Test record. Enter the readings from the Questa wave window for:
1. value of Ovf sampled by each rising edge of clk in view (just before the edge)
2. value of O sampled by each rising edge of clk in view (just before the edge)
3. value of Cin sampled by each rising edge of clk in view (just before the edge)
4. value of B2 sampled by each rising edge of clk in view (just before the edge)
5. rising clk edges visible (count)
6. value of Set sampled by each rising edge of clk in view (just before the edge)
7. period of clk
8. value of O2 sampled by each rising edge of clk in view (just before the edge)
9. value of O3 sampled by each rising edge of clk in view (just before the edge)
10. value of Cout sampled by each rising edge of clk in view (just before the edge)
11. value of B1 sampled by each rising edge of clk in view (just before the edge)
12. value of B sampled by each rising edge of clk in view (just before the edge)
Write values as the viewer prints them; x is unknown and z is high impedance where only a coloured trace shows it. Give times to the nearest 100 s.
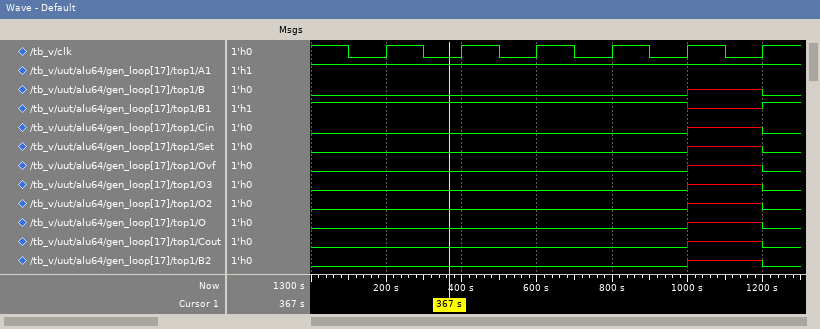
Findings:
0 0 0 0 0 x
0 0 0 0 0 x
0 0 0 0 0 x
0 0 0 0 0 x
6
0 0 0 0 0 x
200 s
0 0 0 0 0 x
0 0 0 0 0 x
0 0 0 0 0 x
1 1 1 1 1 x
0 0 0 0 0 x
